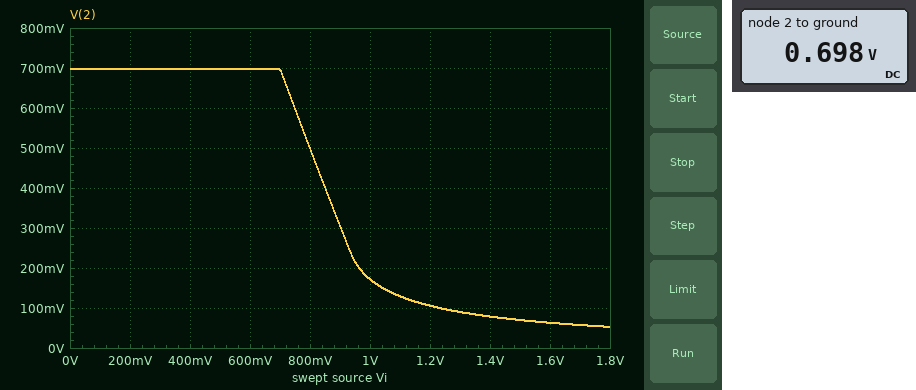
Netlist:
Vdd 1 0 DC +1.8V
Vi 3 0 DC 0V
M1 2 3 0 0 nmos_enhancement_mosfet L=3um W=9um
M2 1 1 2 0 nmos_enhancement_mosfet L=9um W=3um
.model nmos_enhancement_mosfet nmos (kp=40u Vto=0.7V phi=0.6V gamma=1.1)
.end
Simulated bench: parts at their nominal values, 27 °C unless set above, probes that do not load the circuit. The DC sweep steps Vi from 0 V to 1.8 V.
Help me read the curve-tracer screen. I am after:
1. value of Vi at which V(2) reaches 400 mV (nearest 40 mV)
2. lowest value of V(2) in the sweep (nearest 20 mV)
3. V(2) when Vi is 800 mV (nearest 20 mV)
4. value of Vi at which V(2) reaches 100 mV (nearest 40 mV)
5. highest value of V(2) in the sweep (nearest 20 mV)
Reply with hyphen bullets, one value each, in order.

- 840 mV
- 60 mV
- 500 mV
- 1.24 V
- 700 mV
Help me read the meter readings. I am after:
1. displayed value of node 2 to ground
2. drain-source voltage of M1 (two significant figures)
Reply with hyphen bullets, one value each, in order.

- 0.698 V
- 700 mV
